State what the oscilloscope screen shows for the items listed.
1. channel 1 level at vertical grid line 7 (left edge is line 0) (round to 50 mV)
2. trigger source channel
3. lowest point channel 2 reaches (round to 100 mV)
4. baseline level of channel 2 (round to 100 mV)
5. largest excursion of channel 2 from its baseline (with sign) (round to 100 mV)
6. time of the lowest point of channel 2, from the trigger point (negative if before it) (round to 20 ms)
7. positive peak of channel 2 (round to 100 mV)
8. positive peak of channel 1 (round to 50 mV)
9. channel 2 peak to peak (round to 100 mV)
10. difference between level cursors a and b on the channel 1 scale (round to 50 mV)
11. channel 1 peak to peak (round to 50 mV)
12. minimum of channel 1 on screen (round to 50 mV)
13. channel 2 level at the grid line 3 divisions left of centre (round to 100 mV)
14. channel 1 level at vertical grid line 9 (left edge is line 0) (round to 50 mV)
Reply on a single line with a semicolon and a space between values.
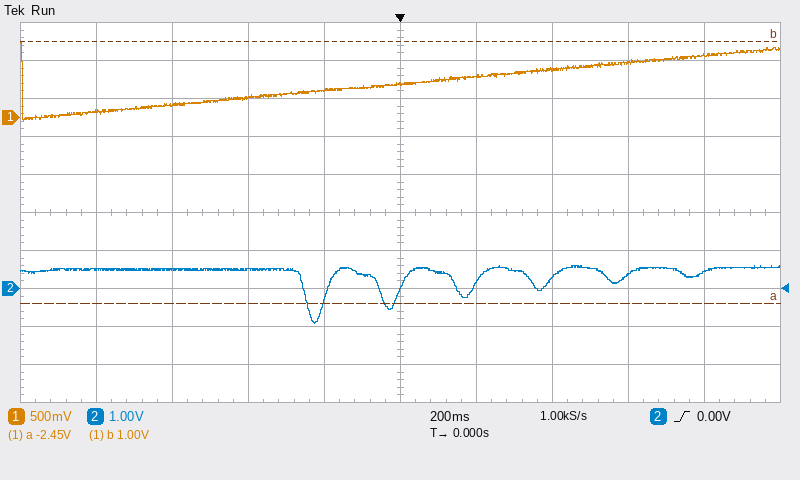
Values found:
650 mV; channel 2; -900 mV; 500 mV; -1.4 V; -220 ms; 600 mV; 1.00 V; 1.5 V; 3.45 V; 1.05 V; -50 mV; 500 mV; 800 mV
